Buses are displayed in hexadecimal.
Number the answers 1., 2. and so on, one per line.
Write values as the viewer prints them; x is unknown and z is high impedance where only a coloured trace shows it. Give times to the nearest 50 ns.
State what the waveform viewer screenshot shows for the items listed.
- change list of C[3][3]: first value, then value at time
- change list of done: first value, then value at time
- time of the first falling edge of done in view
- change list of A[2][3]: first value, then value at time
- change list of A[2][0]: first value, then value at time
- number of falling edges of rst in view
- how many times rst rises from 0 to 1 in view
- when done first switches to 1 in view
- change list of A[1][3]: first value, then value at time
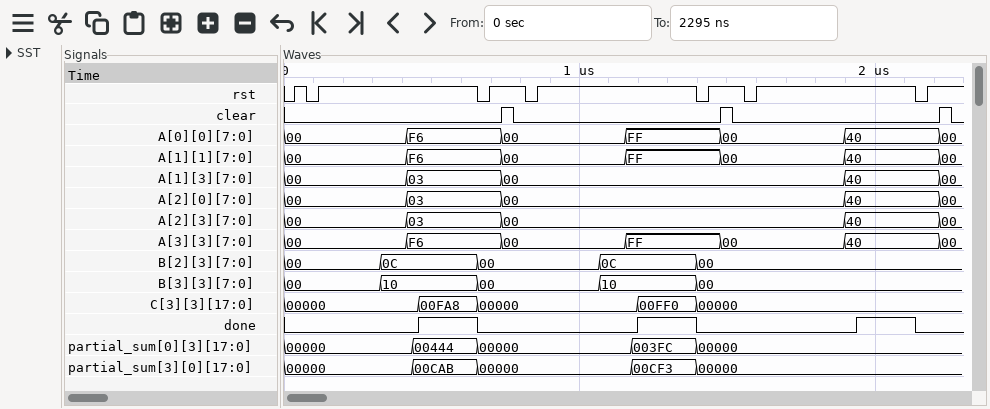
1. 00000, 00FA8 at 450 ns, 00000 at 650 ns, 00FF0 at 1200 ns, 00000 at 1400 ns
2. 0, 1 at 450 ns, 0 at 650 ns, 1 at 1200 ns, 0 at 1400 ns, 1 at 1950 ns, 0 at 2150 ns
3. 650 ns
4. 00, 03 at 400 ns, 00 at 750 ns, 40 at 1900 ns, 00 at 2200 ns
5. 00, 03 at 400 ns, 00 at 750 ns, 40 at 1900 ns, 00 at 2200 ns
6. 6
7. 7
8. 450 ns
9. 00, 03 at 400 ns, 00 at 750 ns, 40 at 1900 ns, 00 at 2200 ns
